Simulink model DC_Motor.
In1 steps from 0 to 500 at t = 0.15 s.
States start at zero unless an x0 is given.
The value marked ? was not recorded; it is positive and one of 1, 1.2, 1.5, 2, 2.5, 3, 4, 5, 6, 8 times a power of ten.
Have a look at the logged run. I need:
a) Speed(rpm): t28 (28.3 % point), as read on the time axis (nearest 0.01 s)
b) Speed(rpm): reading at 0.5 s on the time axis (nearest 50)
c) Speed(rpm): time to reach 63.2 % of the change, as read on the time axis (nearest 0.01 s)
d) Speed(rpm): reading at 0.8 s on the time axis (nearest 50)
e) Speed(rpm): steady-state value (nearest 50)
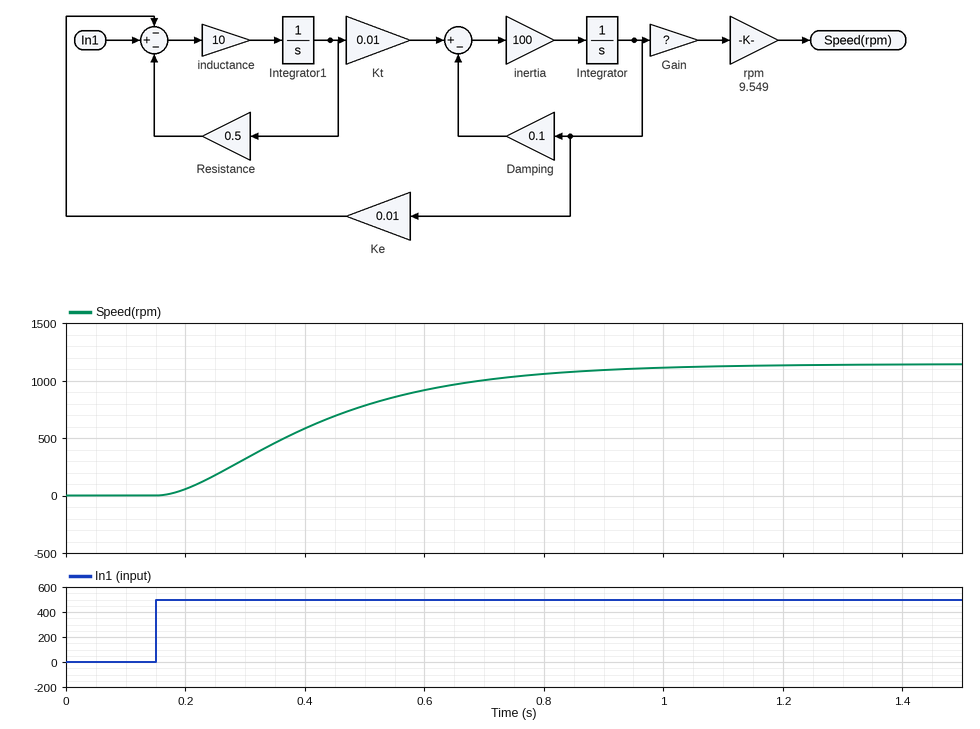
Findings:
0.30 s
800
0.47 s
1050
1150
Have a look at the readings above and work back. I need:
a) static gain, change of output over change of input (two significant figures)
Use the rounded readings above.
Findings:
2.3
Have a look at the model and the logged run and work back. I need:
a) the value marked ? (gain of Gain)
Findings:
1.2
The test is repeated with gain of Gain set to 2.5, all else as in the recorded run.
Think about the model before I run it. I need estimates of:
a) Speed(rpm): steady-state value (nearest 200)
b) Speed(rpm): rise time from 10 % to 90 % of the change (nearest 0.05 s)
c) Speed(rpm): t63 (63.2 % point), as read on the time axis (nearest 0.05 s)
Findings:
2400
0.50 s
0.45 s
